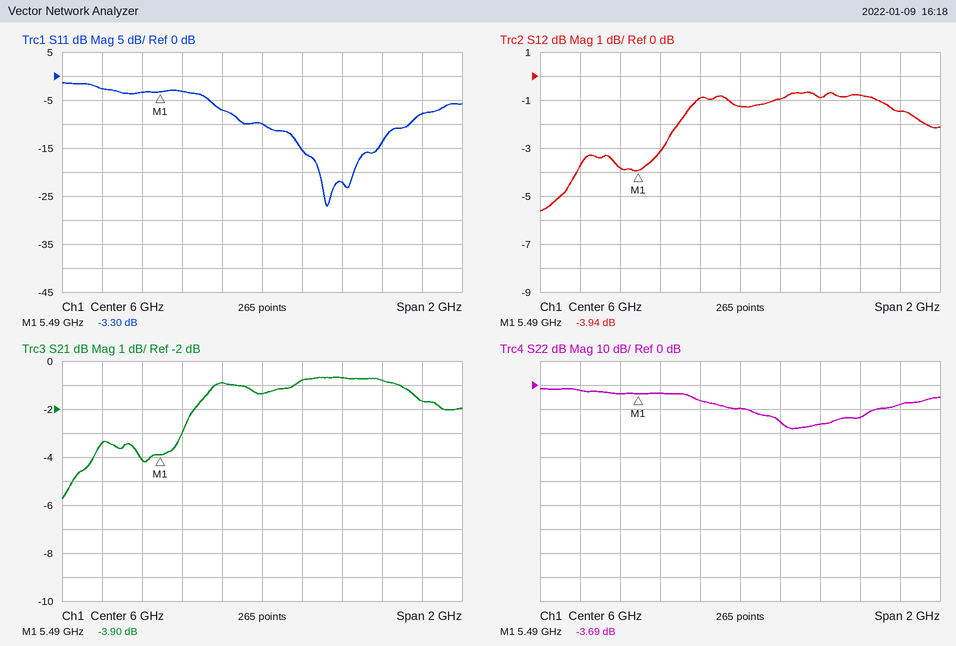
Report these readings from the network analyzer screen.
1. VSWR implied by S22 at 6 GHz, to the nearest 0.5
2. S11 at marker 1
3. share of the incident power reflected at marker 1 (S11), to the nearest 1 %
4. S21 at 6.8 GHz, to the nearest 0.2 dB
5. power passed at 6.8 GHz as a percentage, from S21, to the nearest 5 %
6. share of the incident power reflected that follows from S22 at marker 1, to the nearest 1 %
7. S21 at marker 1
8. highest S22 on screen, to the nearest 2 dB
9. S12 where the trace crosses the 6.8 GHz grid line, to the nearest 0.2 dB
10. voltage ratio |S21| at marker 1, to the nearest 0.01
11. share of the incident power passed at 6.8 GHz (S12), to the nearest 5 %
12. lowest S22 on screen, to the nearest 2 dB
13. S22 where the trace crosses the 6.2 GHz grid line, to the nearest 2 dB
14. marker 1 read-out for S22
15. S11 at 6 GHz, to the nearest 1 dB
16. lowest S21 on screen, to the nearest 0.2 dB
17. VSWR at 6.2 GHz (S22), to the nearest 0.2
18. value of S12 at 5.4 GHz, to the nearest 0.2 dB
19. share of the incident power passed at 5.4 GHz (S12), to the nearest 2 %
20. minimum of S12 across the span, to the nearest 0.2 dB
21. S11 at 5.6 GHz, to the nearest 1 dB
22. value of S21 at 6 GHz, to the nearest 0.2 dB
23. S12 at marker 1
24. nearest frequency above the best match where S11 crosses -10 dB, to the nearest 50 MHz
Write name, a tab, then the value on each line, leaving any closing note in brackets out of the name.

VSWR implied by S22 at 6 GHz, to the nearest 0.5	2.0
S11 at marker 1	-3.30 dB
share of the incident power reflected at marker 1 (S11), to the nearest 1 %	47 %
S21 at 6.8 GHz, to the nearest 0.2 dB	-1.6 dB
power passed at 6.8 GHz as a percentage, from S21, to the nearest 5 %	70 %
share of the incident power reflected that follows from S22 at marker 1, to the nearest 1 %	43 %
S21 at marker 1	-3.90 dB
highest S22 on screen, to the nearest 2 dB	-2 dB
S12 where the trace crosses the 6.8 GHz grid line, to the nearest 0.2 dB	-1.4 dB
voltage ratio |S21| at marker 1, to the nearest 0.01	0.64
share of the incident power passed at 6.8 GHz (S12), to the nearest 5 %	70 %
lowest S22 on screen, to the nearest 2 dB	-18 dB
S22 where the trace crosses the 6.2 GHz grid line, to the nearest 2 dB	-16 dB
marker 1 read-out for S22	-3.69 dB
S11 at 6 GHz, to the nearest 1 dB	-10 dB
lowest S21 on screen, to the nearest 0.2 dB	-5.8 dB
VSWR at 6.2 GHz (S22), to the nearest 0.2	1.4
value of S12 at 5.4 GHz, to the nearest 0.2 dB	-3.8 dB
share of the incident power passed at 5.4 GHz (S12), to the nearest 2 %	42 %
minimum of S12 across the span, to the nearest 0.2 dB	-5.6 dB
S11 at 5.6 GHz, to the nearest 1 dB	-3 dB
value of S21 at 6 GHz, to the nearest 0.2 dB	-1.4 dB
S12 at marker 1	-3.94 dB
nearest frequency above the best match where S11 crosses -10 dB, to the nearest 50 MHz	6.75 GHz
